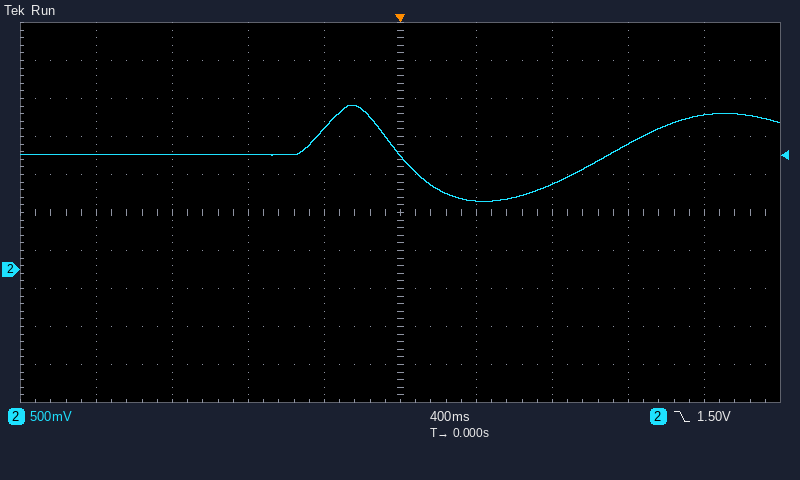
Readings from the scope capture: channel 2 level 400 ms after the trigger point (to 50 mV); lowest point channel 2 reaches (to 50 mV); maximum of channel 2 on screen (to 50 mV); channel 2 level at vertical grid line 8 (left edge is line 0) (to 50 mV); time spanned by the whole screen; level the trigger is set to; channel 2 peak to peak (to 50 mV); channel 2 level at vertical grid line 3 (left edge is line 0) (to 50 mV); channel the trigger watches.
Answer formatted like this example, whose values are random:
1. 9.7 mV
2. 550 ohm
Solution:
1. 900 mV
2. 900 mV
3. 2.15 V
4. 1.65 V
5. 4 s
6. 1.50 V
7. 1.25 V
8. 1.50 V
9. channel 2
